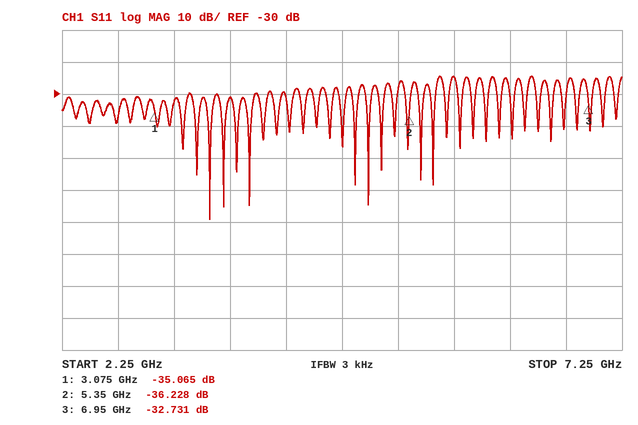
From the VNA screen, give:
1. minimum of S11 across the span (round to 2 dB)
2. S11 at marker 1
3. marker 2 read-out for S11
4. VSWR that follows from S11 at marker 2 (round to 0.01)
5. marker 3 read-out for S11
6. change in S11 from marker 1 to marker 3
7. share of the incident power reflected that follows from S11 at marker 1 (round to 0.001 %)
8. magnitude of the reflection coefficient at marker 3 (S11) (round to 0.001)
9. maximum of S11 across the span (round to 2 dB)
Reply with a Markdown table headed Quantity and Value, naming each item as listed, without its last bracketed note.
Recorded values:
| Quantity | Value |
|---|---|
| minimum of S11 across the span | -70 dB |
| S11 at marker 1 | -35.065 dB |
| marker 2 read-out for S11 | -36.228 dB |
| VSWR that follows from S11 at marker 2 | 1.03 |
| marker 3 read-out for S11 | -32.731 dB |
| change in S11 from marker 1 to marker 3 | 2.334 dB |
| share of the incident power reflected that follows from S11 at marker 1 | 0.031 % |
| magnitude of the reflection coefficient at marker 3 (S11) | 0.023 |
| maximum of S11 across the span | -24 dB |
